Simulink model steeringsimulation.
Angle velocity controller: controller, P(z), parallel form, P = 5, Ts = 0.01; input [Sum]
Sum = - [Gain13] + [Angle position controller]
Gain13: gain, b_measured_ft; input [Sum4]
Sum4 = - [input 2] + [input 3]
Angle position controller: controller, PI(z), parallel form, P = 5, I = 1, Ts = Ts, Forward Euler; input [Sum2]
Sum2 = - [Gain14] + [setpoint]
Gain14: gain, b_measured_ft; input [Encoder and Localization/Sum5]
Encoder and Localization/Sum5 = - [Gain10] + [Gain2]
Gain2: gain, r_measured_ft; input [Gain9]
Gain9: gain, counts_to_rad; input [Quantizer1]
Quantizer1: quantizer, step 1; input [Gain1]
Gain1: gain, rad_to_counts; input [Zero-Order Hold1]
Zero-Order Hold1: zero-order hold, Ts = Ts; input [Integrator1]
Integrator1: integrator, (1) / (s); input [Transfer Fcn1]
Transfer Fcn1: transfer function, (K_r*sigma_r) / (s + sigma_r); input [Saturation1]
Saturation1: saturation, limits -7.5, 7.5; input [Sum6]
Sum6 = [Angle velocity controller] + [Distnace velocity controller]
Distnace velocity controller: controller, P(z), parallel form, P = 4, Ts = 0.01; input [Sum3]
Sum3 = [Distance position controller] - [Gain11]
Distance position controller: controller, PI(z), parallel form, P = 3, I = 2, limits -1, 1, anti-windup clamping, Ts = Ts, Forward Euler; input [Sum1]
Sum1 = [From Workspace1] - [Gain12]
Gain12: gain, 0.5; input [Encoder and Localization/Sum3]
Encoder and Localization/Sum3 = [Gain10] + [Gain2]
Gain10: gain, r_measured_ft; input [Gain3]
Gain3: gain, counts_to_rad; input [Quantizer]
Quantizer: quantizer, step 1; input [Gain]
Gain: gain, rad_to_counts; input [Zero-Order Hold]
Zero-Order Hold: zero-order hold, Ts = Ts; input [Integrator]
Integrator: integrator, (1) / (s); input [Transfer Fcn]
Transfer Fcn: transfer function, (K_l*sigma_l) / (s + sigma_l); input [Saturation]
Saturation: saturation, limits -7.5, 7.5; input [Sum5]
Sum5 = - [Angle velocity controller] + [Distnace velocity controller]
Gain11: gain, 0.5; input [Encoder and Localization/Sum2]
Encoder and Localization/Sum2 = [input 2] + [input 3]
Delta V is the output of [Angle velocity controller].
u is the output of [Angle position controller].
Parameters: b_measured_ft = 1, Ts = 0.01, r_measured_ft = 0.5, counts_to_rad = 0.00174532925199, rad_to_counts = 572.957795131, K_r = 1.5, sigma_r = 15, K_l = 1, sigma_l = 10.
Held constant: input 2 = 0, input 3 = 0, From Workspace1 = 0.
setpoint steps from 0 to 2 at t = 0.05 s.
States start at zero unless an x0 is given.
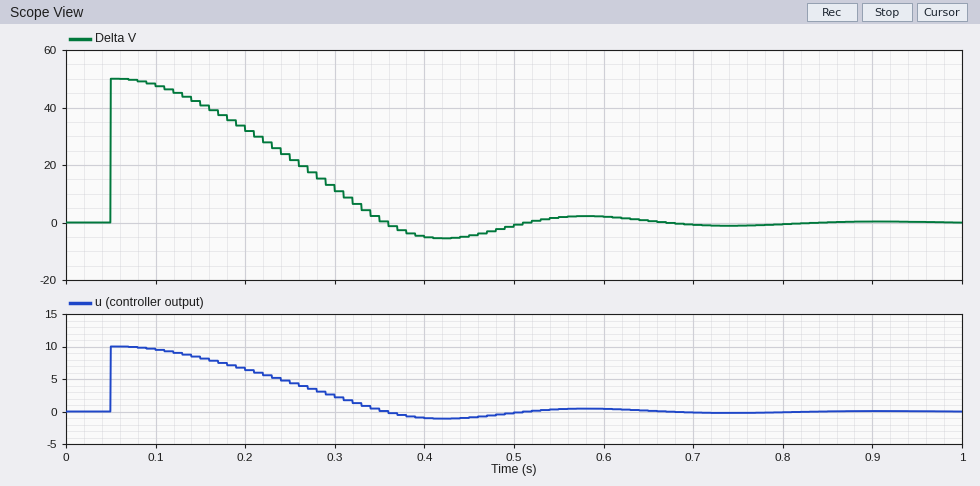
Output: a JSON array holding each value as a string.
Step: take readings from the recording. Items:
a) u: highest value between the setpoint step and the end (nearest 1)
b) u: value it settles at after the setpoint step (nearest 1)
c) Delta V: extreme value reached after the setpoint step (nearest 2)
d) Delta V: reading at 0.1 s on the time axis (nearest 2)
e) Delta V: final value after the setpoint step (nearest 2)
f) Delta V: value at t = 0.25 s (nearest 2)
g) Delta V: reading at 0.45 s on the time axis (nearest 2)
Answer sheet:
["10", "0", "50", "48", "0", "22", "-4"]
